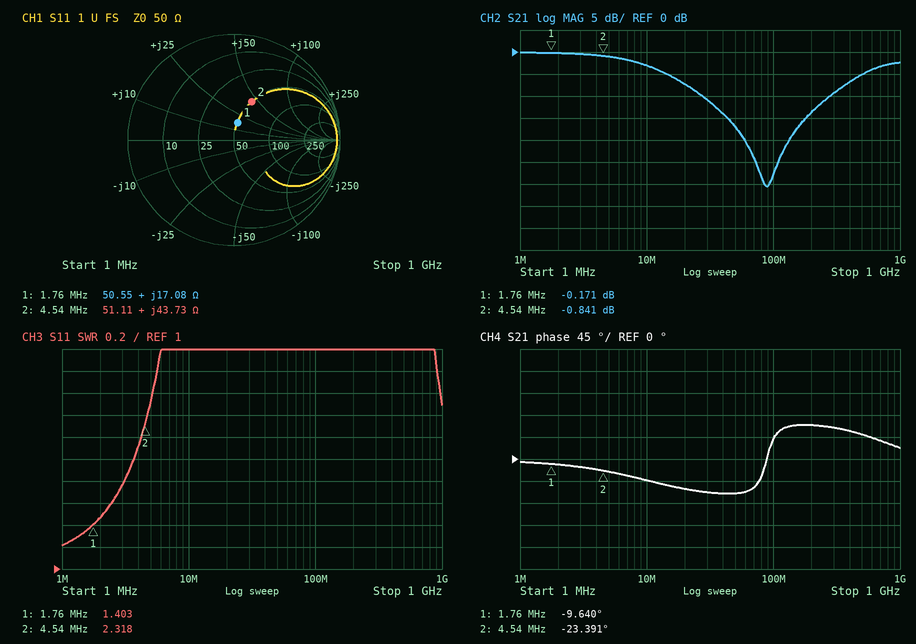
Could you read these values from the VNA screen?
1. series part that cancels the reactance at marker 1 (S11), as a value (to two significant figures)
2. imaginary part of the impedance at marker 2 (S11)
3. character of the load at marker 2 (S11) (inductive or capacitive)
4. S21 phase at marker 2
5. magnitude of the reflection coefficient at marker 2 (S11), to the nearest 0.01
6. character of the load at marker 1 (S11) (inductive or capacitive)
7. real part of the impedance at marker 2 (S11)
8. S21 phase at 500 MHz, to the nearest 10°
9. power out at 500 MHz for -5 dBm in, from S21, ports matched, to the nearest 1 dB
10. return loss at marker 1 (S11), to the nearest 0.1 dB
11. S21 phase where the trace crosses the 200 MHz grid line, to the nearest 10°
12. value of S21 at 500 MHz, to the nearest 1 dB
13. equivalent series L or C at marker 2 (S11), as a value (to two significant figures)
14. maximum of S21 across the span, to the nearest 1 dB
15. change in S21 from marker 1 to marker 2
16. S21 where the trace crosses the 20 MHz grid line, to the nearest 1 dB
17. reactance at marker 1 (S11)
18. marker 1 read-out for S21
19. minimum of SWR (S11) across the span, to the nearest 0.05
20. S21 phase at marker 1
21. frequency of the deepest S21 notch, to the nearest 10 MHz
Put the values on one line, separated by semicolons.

5.3 nF; +43.73 Ω; inductive; -23.391°; 0.40; inductive; 51.11 Ω; 50°; -10 dBm; 15.5 dB; 70°; -5 dB; 1.5 µH; 0 dB; -0.670 dB; -7 dB; +17.08 Ω; -0.171 dB; 1.20; -9.640°; 90 MHz
